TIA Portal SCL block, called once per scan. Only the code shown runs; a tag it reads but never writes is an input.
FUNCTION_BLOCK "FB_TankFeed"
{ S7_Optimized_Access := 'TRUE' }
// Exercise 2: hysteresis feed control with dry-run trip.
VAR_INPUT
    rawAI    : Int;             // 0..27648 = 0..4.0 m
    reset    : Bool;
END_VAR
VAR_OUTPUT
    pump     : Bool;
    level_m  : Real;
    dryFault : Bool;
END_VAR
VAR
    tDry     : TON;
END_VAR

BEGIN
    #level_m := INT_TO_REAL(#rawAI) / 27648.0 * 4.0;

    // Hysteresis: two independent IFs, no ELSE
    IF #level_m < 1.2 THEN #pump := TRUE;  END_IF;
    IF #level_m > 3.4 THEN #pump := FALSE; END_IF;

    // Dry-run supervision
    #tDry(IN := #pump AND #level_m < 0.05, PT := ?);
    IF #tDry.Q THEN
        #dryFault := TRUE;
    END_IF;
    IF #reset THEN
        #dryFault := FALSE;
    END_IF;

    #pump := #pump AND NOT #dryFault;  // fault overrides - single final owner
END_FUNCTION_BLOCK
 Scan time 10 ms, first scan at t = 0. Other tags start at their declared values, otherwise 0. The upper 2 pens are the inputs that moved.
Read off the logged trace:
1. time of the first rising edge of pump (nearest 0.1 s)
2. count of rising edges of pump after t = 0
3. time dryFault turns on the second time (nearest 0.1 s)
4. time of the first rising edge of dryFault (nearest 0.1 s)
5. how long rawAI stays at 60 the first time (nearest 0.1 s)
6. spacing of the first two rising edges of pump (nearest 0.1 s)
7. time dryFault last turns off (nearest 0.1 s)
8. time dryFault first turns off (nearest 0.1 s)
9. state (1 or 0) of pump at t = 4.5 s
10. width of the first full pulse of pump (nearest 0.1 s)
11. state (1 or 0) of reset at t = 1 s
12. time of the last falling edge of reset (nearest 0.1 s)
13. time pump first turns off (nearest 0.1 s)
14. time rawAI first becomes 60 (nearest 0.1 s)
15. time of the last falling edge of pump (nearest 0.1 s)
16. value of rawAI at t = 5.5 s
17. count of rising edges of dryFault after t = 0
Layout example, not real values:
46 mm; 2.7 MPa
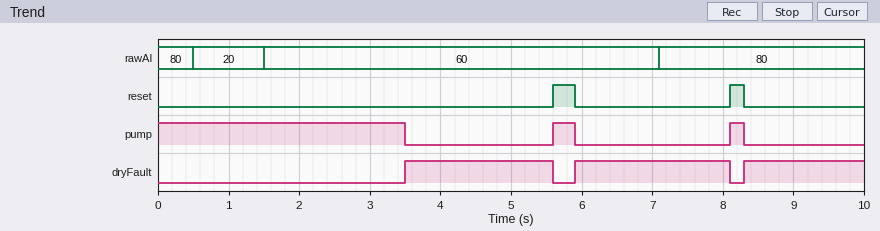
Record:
5.6 s; 2; 5.9 s; 3.5 s; 5.6 s; 2.5 s; 8.1 s; 5.6 s; 0; 0.3 s; 0; 8.3 s; 3.5 s; 1.5 s; 8.3 s; 60; 3
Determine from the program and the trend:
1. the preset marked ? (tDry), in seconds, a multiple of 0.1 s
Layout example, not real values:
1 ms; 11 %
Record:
3.5 s
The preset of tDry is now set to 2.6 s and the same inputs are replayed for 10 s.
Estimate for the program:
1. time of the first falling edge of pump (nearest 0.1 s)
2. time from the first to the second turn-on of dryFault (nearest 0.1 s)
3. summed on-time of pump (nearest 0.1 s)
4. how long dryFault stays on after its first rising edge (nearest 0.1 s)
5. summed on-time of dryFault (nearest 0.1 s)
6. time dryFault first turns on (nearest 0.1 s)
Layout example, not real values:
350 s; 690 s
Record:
2.6 s; 3.3 s; 3.1 s; 3.0 s; 6.9 s; 2.6 s
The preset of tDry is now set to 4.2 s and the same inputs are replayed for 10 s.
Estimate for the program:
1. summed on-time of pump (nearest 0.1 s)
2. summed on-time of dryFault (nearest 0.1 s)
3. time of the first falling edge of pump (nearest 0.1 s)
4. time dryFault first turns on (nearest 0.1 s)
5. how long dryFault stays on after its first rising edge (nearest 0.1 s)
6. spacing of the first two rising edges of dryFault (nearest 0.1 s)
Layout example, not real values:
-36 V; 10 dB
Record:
4.7 s; 5.3 s; 4.2 s; 4.2 s; 1.4 s; 1.7 s
